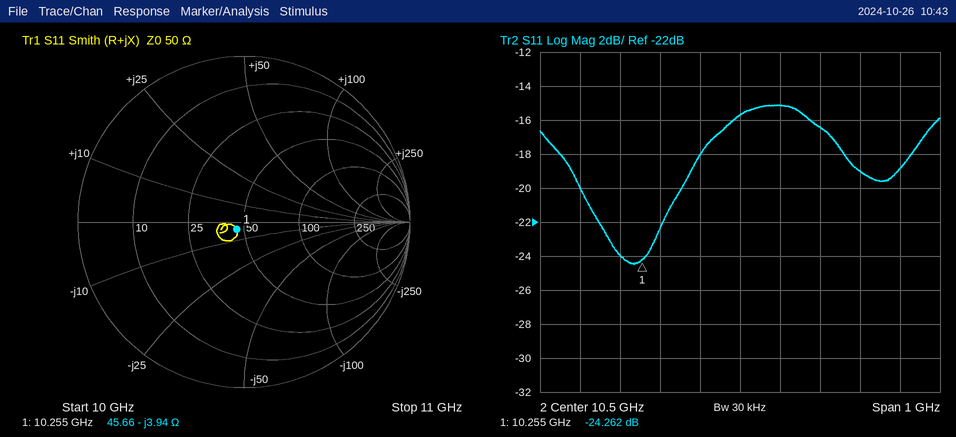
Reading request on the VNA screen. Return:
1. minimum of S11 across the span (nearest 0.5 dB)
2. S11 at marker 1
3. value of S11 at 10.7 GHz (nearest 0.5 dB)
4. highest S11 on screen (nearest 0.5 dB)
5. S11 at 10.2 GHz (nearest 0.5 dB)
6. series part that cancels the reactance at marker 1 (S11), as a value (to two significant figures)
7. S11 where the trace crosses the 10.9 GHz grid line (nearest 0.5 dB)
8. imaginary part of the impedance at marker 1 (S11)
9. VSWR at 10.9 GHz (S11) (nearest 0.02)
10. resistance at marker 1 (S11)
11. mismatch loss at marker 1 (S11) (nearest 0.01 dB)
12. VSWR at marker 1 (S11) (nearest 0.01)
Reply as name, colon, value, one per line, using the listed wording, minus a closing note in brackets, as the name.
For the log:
minimum of S11 across the span: -24.5 dB
S11 at marker 1: -24.262 dB
value of S11 at 10.7 GHz: -16.5 dB
highest S11 on screen: -15.0 dB
S11 at 10.2 GHz: -24.0 dB
series part that cancels the reactance at marker 1 (S11), as a value: 61 pH
S11 where the trace crosses the 10.9 GHz grid line: -19.0 dB
imaginary part of the impedance at marker 1: -3.94 Ω
VSWR at 10.9 GHz (S11): 1.26
resistance at marker 1: 45.66 Ω
mismatch loss at marker 1 (S11): 0.02 dB
VSWR at marker 1 (S11): 1.13
